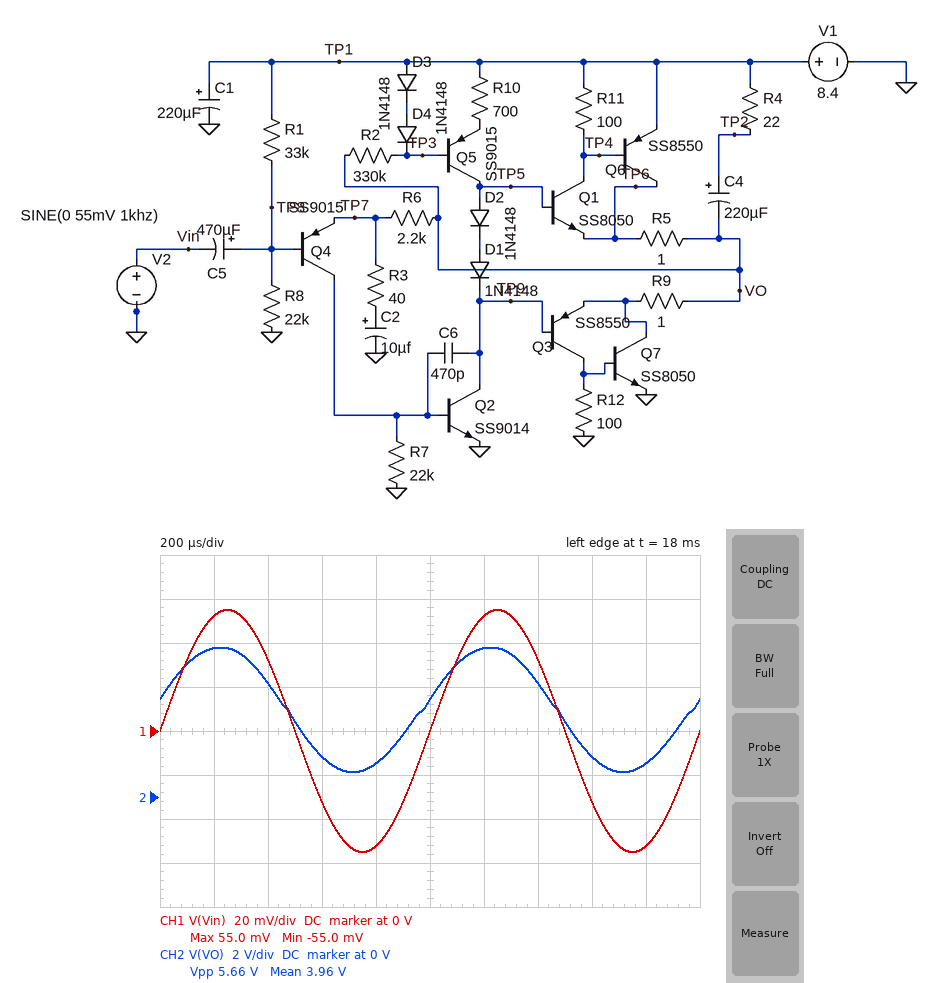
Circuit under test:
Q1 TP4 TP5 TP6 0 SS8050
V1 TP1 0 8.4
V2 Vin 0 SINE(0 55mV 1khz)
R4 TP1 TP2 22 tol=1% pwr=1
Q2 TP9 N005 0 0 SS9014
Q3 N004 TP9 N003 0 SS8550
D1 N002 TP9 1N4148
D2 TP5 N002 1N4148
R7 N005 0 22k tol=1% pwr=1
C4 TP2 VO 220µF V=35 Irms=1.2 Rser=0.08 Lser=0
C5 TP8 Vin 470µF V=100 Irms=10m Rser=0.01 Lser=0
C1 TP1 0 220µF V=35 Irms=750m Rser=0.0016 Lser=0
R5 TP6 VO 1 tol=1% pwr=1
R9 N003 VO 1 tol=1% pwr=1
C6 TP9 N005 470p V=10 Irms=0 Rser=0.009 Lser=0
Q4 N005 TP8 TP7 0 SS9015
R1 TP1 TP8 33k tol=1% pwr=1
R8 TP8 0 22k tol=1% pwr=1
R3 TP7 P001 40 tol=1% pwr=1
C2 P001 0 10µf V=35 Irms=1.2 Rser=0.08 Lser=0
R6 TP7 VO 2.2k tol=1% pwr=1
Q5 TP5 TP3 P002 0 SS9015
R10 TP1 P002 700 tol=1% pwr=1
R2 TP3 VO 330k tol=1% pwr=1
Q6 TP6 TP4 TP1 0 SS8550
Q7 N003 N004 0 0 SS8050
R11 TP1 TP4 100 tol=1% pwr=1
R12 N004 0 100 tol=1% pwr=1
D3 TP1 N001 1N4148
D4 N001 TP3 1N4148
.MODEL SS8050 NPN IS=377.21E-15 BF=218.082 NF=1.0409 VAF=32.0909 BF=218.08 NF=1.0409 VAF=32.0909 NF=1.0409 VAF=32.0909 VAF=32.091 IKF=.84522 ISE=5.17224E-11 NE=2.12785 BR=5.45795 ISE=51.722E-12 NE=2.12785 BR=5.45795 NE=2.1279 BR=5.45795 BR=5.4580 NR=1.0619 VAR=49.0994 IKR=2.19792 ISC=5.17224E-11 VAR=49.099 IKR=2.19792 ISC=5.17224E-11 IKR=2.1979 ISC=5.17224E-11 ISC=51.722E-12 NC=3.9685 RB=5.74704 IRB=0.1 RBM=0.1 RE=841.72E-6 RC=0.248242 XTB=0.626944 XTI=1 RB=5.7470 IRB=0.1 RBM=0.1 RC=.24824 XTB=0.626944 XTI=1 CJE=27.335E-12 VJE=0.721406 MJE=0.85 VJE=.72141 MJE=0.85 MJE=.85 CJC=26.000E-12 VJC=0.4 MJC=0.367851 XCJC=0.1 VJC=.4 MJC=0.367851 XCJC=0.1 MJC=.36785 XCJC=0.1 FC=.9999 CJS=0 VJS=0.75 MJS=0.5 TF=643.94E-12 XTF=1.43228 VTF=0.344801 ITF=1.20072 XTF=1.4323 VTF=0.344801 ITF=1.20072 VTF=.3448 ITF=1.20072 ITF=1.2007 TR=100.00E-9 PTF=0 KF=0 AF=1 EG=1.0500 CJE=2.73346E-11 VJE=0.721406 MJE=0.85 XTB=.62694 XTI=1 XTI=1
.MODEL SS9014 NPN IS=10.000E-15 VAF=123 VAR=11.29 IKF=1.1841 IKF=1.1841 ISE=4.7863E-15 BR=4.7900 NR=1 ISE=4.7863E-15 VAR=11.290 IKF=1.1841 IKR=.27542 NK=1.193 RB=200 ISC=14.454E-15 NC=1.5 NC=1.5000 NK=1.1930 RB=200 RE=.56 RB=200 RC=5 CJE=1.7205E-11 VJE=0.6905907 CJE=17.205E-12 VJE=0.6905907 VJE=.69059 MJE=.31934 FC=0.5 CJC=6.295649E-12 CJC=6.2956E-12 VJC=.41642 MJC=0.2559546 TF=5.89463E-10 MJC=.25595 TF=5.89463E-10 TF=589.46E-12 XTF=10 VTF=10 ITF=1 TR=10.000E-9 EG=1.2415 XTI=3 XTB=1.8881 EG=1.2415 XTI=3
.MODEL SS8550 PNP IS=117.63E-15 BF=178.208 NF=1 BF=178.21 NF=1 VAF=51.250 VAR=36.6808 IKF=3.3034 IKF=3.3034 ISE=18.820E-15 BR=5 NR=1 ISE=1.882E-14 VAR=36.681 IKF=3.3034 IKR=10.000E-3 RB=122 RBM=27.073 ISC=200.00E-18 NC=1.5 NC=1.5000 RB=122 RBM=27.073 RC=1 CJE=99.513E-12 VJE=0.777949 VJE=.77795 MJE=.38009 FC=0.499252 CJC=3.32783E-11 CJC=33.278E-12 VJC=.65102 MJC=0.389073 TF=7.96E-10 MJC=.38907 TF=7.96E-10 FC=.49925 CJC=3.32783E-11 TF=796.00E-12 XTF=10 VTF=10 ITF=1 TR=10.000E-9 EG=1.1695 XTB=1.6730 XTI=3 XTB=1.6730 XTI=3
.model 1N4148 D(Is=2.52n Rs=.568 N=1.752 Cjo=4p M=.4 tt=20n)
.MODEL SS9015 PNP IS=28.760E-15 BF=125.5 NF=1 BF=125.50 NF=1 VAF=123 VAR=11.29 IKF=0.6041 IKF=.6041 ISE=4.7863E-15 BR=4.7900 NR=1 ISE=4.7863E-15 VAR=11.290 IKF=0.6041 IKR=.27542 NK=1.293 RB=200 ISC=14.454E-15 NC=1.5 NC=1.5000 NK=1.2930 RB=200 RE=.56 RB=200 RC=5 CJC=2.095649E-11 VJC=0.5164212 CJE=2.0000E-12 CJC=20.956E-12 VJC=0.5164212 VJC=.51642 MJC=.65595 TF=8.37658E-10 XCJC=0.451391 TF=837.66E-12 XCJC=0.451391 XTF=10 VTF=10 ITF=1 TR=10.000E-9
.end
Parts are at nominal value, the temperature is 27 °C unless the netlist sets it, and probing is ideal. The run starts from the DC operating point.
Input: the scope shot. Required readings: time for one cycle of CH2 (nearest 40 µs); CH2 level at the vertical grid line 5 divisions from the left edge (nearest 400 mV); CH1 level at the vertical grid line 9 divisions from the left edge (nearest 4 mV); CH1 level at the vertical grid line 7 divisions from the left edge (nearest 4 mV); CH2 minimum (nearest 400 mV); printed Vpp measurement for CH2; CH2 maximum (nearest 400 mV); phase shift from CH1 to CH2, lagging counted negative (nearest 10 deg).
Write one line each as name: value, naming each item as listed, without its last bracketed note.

time for one cycle of CH2: 1.00 ms
CH2 level at the vertical grid line 5 divisions from the left edge: 4.4 V
CH1 level at the vertical grid line 9 divisions from the left edge: -52 mV
CH1 level at the vertical grid line 7 divisions from the left edge: 32 mV
CH2 minimum: 1.2 V
printed Vpp measurement for CH2: 5.66 V
CH2 maximum: 6.8 V
phase shift from CH1 to CH2, lagging counted negative: 10 deg
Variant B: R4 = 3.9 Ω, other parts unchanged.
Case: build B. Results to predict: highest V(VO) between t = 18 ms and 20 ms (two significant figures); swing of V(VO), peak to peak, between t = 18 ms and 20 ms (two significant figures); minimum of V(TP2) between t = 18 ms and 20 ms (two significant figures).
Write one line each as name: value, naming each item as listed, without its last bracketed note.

highest V(VO) between t = 18 ms and 20 ms: 6.5 V
swing of V(VO), peak to peak, between t = 18 ms and 20 ms: 5.0 V
minimum of V(TP2) between t = 18 ms and 20 ms: 5.9 V
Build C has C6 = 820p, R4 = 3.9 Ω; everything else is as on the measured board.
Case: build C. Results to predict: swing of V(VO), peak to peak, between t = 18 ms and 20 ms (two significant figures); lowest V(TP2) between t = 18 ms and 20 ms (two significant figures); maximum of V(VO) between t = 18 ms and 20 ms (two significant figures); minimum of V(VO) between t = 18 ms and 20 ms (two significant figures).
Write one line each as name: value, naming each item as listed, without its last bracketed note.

swing of V(VO), peak to peak, between t = 18 ms and 20 ms: 5.0 V
lowest V(TP2) between t = 18 ms and 20 ms: 5.9 V
maximum of V(VO) between t = 18 ms and 20 ms: 6.5 V
minimum of V(VO) between t = 18 ms and 20 ms: 1.5 V
